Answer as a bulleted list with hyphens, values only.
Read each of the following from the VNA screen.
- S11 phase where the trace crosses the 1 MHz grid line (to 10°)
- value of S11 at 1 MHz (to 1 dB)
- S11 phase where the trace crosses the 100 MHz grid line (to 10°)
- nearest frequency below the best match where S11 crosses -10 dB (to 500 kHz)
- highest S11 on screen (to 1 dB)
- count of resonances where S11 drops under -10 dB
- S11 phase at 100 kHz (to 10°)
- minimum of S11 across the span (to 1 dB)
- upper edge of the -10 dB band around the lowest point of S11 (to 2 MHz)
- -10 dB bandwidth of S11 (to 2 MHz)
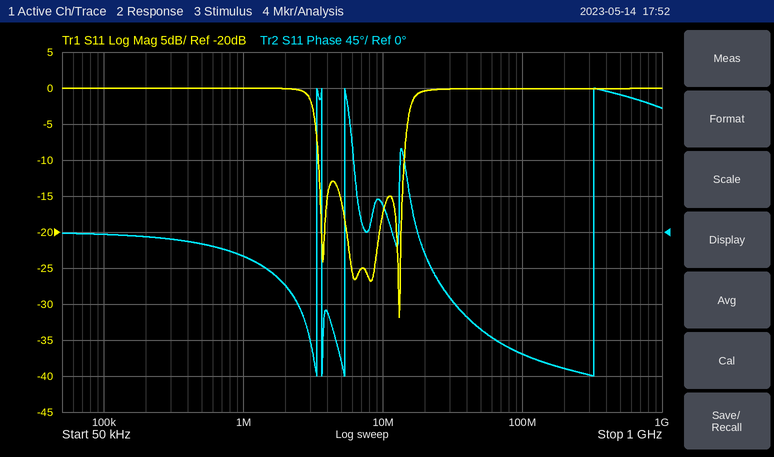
- -30°
- 0 dB
- -150°
- 3.5 MHz
- 0 dB
- 3
- 0°
- -32 dB
- 14 MHz
- 10 MHz
